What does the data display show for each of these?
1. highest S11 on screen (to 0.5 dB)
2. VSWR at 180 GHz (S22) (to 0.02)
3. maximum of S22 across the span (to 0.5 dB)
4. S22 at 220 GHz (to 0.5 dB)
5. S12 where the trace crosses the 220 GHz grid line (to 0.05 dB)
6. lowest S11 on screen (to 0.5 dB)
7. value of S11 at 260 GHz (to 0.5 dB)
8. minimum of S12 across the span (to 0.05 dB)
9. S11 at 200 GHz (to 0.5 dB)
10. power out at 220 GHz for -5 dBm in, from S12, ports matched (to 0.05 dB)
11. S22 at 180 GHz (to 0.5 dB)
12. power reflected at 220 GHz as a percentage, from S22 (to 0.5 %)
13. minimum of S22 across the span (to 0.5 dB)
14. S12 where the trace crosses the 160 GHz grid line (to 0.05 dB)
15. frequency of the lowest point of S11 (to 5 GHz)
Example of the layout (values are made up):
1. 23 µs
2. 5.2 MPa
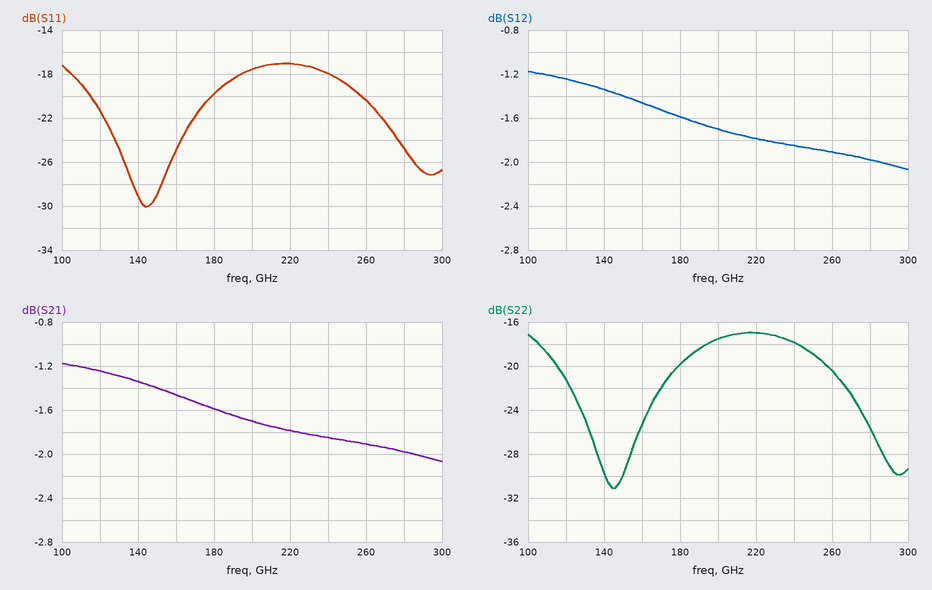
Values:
1. -17.0 dB
2. 1.22
3. -17.0 dB
4. -17.0 dB
5. -1.80 dB
6. -30.0 dB
7. -20.5 dB
8. -2.05 dB
9. -17.5 dB
10. -6.80 dBm
11. -20.0 dB
12. 2.0 %
13. -31.0 dB
14. -1.45 dB
15. 145 GHz
